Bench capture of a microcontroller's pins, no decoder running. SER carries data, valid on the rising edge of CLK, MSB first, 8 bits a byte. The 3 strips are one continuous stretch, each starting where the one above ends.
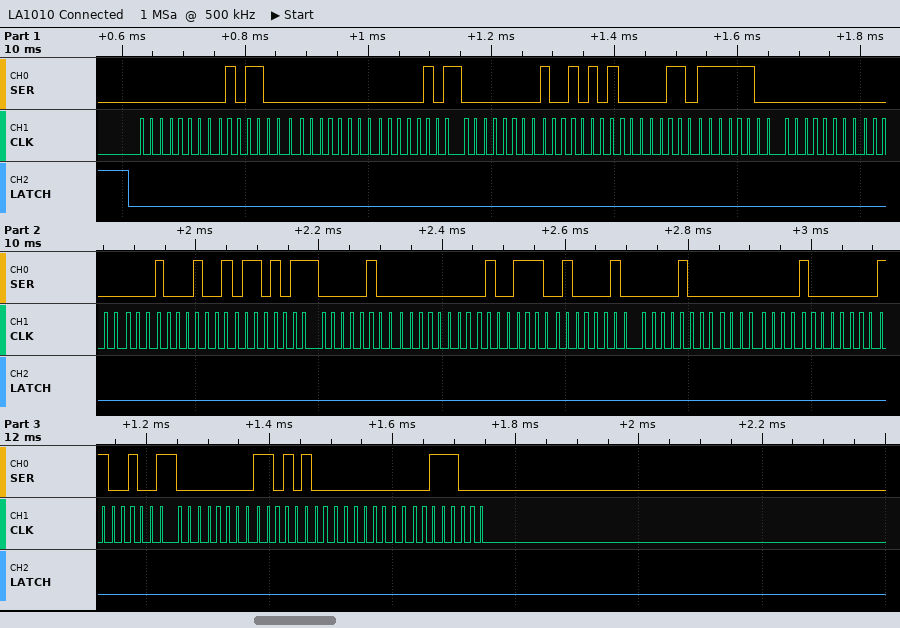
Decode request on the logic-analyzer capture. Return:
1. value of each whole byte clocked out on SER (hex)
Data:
00 58 00 05 00 95 06 FC 00 00 89 6B 04 00 4E 42 08 00 80 C9 00 D4 00 38
